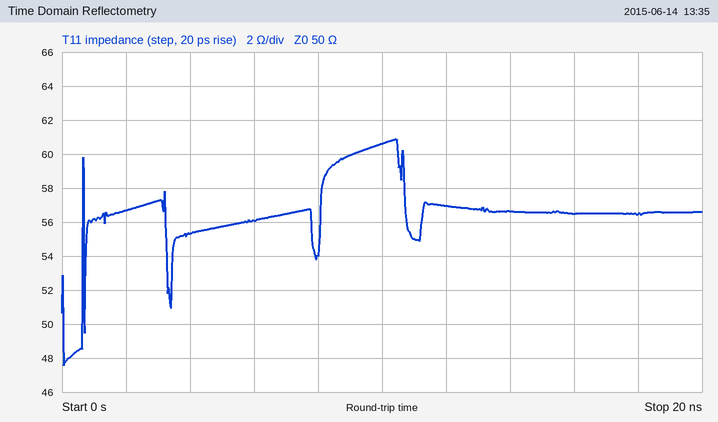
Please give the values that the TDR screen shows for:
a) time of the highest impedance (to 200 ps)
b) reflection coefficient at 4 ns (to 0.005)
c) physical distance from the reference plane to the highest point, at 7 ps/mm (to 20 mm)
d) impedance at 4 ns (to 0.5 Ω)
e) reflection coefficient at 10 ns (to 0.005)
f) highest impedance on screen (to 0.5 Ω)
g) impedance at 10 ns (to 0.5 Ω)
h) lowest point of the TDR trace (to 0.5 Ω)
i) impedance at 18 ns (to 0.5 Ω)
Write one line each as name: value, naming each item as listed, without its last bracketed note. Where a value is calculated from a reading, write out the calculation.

time of the highest impedance: 10.4 ns
reflection coefficient at 4 ns: (55.5 − 50)/(55.5 + 50) ≈ +0.0521, so +0.050 to the nearest 0.005
physical distance from the reference plane to the highest point, at 7 ps/mm: 10.4 ns / 2 / 7 ps/mm ≈ 743 mm, so 740 mm to the nearest 20 mm
impedance at 4 ns: 55.5 Ω
reflection coefficient at 10 ns: (60.5 − 50)/(60.5 + 50) ≈ +0.095
highest impedance on screen: 61.0 Ω
impedance at 10 ns: 60.5 Ω
lowest point of the TDR trace: 47.5 Ω
impedance at 18 ns: 56.5 Ω
